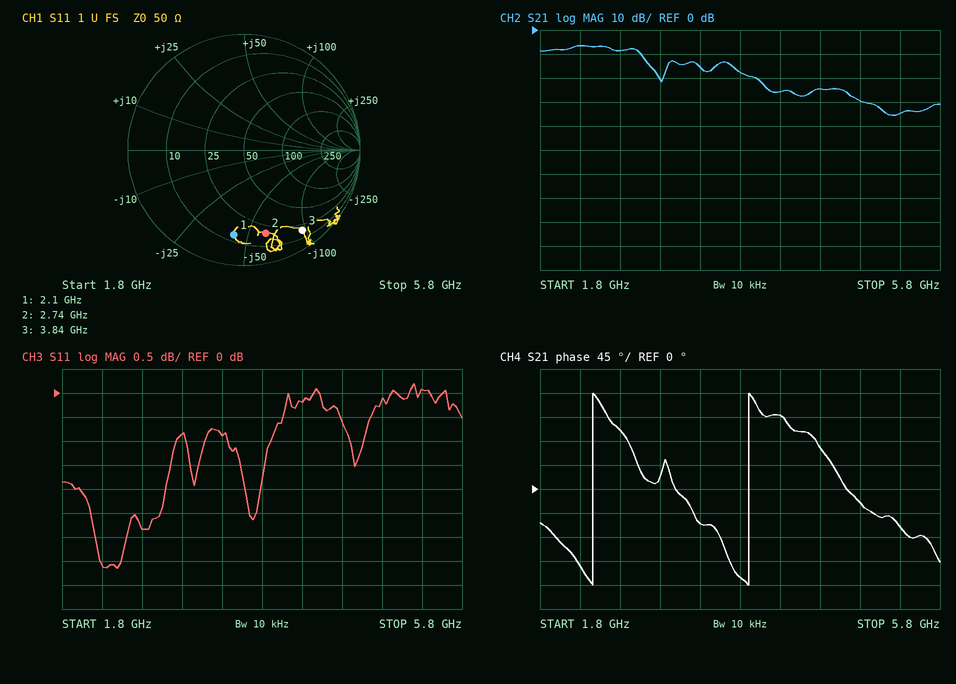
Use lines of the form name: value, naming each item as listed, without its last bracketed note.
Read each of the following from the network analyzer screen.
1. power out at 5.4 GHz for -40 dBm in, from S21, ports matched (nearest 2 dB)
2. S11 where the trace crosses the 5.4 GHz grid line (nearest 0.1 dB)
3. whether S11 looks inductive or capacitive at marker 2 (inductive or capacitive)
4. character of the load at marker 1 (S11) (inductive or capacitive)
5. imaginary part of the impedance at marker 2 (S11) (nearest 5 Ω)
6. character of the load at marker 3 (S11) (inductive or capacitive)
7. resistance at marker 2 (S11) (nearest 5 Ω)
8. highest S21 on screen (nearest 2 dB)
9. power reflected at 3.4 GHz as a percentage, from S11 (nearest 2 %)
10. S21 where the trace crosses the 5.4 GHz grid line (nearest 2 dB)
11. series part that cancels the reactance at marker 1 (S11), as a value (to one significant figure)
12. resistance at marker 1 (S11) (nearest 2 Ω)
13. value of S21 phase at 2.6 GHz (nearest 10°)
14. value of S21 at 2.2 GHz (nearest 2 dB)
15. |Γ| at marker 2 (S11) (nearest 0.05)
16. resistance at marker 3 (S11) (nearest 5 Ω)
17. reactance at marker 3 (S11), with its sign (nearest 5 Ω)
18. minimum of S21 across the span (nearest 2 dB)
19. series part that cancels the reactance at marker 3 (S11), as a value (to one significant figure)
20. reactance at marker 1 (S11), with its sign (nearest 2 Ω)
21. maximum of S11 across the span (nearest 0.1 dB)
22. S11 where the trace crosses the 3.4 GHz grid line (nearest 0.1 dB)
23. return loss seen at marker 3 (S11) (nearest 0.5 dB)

power out at 5.4 GHz for -40 dBm in, from S21, ports matched: -74 dBm
S11 where the trace crosses the 5.4 GHz grid line: 0.1 dB
whether S11 looks inductive or capacitive at marker 2: capacitive
character of the load at marker 1 (S11): capacitive
imaginary part of the impedance at marker 2 (S11): -60 Ω
character of the load at marker 3 (S11): capacitive
resistance at marker 2 (S11): 20 Ω
highest S21 on screen: -6 dB
power reflected at 3.4 GHz as a percentage, from S11: 82 %
S21 where the trace crosses the 5.4 GHz grid line: -34 dB
series part that cancels the reactance at marker 1 (S11), as a value: 3 nH
resistance at marker 1 (S11): 14 Ω
value of S21 phase at 2.6 GHz: 110°
value of S21 at 2.2 GHz: -6 dB
|Γ| at marker 2 (S11): 0.75
resistance at marker 3 (S11): 20 Ω
reactance at marker 3 (S11), with its sign: -95 Ω
minimum of S21 across the span: -36 dB
series part that cancels the reactance at marker 3 (S11), as a value: 4 nH
reactance at marker 1 (S11), with its sign: -42 Ω
maximum of S11 across the span: 0.2 dB
S11 where the trace crosses the 3.4 GHz grid line: -0.9 dB
return loss seen at marker 3 (S11): 1.5 dB
